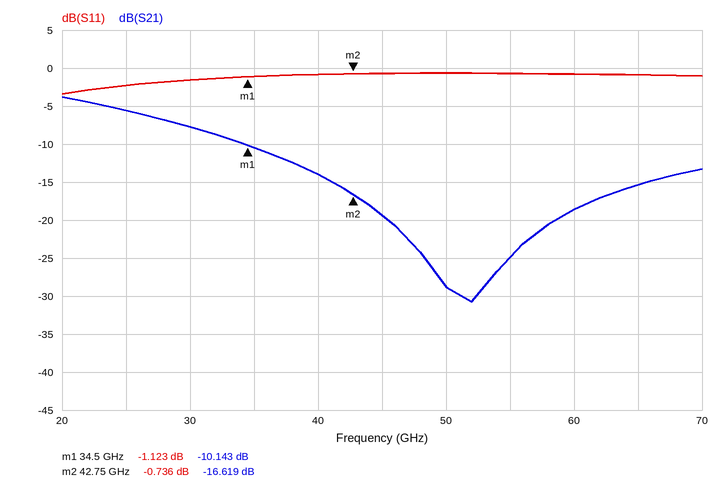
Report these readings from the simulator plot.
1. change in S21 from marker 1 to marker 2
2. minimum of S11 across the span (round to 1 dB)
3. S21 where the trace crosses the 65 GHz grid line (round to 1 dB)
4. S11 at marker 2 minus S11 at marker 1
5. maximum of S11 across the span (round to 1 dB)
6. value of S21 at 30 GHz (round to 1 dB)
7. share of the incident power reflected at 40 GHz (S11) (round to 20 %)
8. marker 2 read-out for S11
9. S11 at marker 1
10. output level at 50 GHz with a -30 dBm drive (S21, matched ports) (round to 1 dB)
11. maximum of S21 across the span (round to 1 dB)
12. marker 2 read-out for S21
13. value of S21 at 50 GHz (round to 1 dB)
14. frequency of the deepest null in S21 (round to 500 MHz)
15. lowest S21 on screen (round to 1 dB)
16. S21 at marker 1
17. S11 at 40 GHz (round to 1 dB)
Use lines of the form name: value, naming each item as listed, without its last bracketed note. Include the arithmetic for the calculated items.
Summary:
change in S21 from marker 1 to marker 2: -16.619 − (-10.143) = -6.476 dB
minimum of S11 across the span: -3 dB
S21 where the trace crosses the 65 GHz grid line: -15 dB
S11 at marker 2 minus S11 at marker 1: -0.736 − (-1.123) = 0.387 dB
maximum of S11 across the span: -1 dB
value of S21 at 30 GHz: -8 dB
share of the incident power reflected at 40 GHz (S11): 10^(-1/10) ≈ 79.4 %, so 80 % to the nearest 20 %
marker 2 read-out for S11: -0.736 dB
S11 at marker 1: -1.123 dB
output level at 50 GHz with a -30 dBm drive (S21, matched ports): -30 dBm + (-29 dB) = -59 dBm
maximum of S21 across the span: -4 dB
marker 2 read-out for S21: -16.619 dB
value of S21 at 50 GHz: -29 dB
frequency of the deepest null in S21: 52.0 GHz
lowest S21 on screen: -31 dB
S21 at marker 1: -10.143 dB
S11 at 40 GHz: -1 dB
